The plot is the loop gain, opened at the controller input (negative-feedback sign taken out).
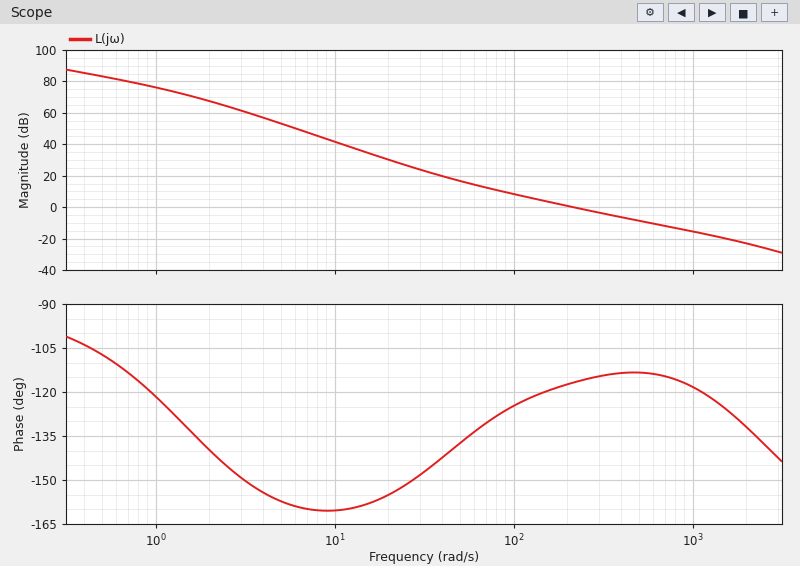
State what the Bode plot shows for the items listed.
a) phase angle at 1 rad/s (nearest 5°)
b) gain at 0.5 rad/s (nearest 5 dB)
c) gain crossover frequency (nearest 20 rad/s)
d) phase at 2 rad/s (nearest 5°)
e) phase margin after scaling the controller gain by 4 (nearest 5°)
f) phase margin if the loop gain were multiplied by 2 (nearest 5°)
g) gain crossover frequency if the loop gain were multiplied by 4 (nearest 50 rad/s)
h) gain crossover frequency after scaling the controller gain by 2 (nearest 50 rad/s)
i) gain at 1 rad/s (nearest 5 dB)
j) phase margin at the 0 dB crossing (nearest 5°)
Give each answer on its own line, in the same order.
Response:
-120°
85 dB
220 rad/s
-140°
65°
65°
700 rad/s
400 rad/s
75 dB
65°
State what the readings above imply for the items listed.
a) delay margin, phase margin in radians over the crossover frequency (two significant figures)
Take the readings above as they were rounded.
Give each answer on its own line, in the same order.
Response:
0.0052 s
